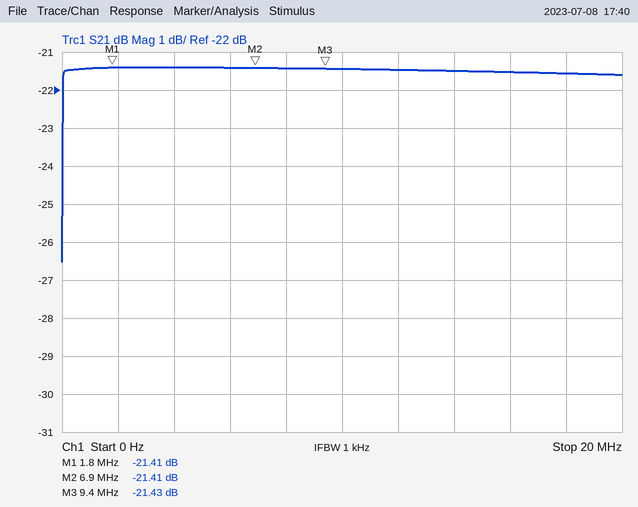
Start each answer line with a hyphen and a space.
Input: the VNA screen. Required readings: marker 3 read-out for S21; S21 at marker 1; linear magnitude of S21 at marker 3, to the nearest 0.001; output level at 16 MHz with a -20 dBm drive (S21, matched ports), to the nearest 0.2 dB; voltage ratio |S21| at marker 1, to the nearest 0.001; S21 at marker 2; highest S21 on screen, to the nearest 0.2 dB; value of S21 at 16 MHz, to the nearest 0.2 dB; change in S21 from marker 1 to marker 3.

- -21.43 dB
- -21.41 dB
- 0.085
- -41.6 dBm
- 0.085
- -21.41 dB
- -21.4 dB
- -21.6 dB
- -0.02 dB
